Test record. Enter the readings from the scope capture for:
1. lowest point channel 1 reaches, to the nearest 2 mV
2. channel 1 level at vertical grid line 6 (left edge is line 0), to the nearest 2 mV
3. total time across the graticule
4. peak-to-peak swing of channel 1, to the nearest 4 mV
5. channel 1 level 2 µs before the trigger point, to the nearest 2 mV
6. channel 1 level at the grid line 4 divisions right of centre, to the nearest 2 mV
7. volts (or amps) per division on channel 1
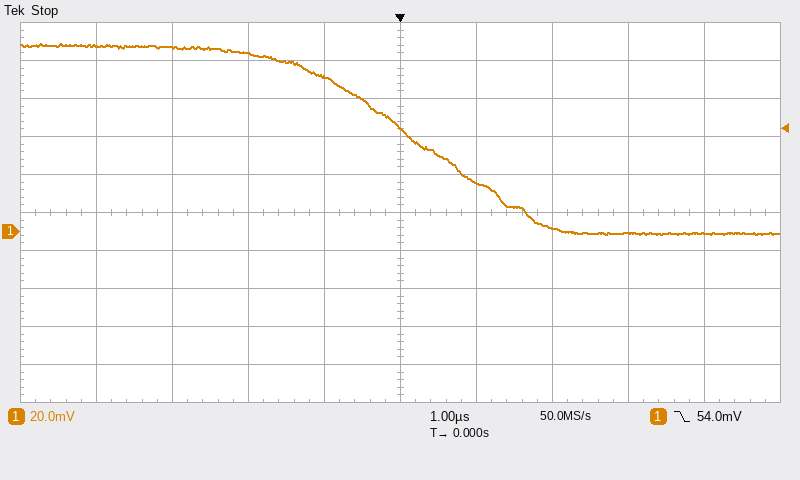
-2 mV
26 mV
10 µs
100 mV
94 mV
0 mV
20 mV
